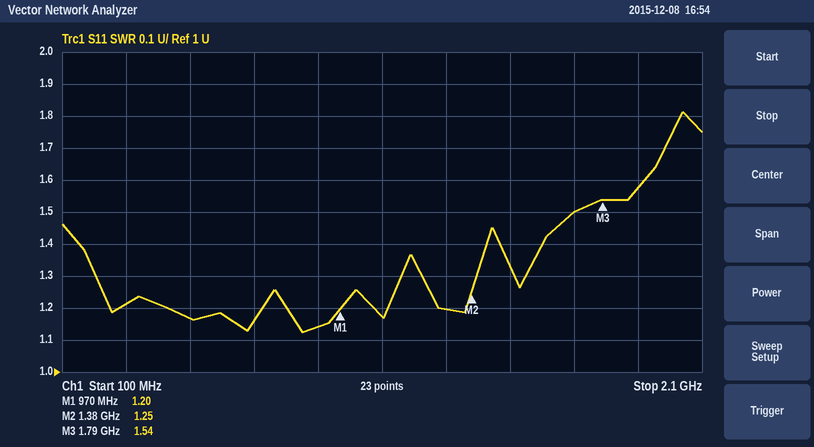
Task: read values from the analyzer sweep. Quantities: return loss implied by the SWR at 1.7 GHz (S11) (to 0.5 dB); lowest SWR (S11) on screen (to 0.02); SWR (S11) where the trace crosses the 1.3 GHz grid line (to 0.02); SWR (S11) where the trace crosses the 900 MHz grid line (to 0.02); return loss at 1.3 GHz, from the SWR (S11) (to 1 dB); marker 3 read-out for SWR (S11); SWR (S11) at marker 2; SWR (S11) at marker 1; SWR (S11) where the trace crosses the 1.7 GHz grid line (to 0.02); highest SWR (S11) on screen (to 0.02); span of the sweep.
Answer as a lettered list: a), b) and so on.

a) 14.0 dB
b) 1.12
c) 1.20
d) 1.14
e) 21 dB
f) 1.54
g) 1.25
h) 1.20
i) 1.50
j) 1.82
k) 2 GHz
